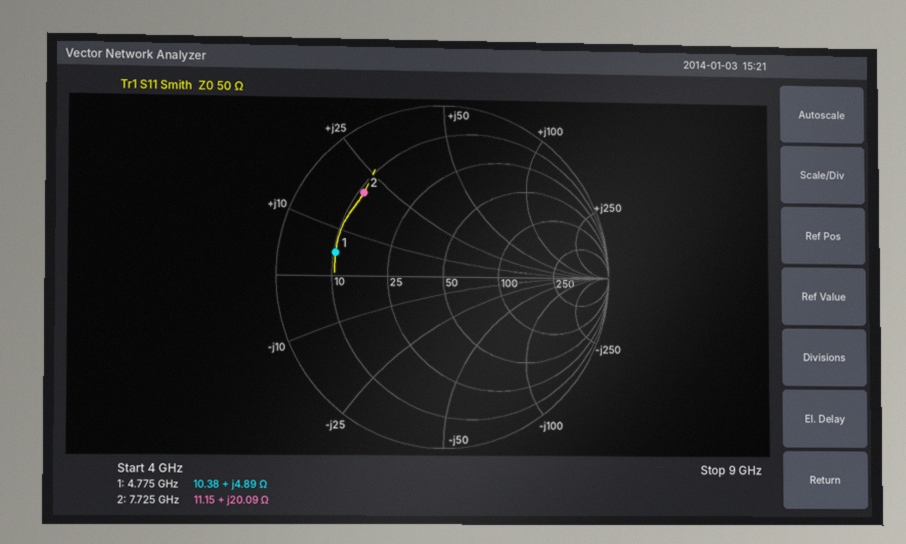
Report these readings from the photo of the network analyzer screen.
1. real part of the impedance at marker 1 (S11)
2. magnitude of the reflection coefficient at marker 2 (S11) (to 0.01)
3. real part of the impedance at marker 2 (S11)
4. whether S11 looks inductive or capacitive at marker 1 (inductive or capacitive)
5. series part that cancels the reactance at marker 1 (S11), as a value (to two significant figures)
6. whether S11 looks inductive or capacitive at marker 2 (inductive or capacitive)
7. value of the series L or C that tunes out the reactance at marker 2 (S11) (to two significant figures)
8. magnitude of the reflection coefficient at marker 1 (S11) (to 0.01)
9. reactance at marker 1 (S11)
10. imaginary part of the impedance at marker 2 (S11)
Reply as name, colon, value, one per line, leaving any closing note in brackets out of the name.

real part of the impedance at marker 1: 10.38 Ω
magnitude of the reflection coefficient at marker 2 (S11): 0.68
real part of the impedance at marker 2: 11.15 Ω
whether S11 looks inductive or capacitive at marker 1: inductive
series part that cancels the reactance at marker 1 (S11), as a value: 6.8 pF
whether S11 looks inductive or capacitive at marker 2: inductive
value of the series L or C that tunes out the reactance at marker 2 (S11): 1.0 pF
magnitude of the reflection coefficient at marker 1 (S11): 0.66
reactance at marker 1: +4.89 Ω
imaginary part of the impedance at marker 2: +20.09 Ω
